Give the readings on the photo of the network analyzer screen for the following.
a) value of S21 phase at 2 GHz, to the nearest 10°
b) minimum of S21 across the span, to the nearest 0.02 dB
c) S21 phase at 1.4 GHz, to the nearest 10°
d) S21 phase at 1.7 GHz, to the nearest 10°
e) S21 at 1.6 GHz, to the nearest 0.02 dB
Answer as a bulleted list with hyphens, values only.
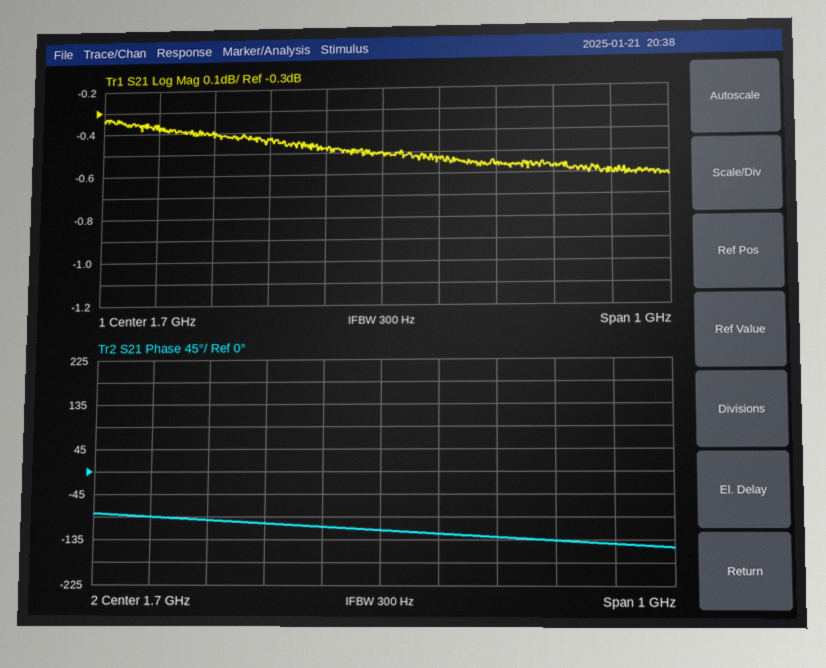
- -140°
- -0.62 dB
- -100°
- -120°
- -0.48 dB
